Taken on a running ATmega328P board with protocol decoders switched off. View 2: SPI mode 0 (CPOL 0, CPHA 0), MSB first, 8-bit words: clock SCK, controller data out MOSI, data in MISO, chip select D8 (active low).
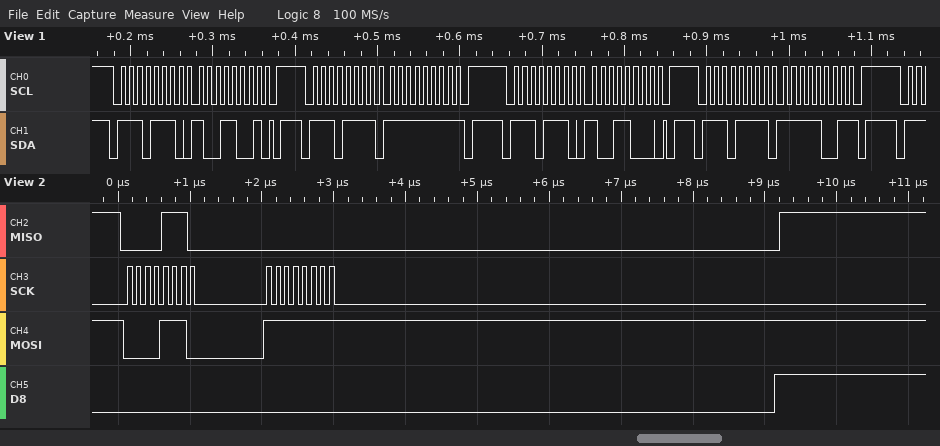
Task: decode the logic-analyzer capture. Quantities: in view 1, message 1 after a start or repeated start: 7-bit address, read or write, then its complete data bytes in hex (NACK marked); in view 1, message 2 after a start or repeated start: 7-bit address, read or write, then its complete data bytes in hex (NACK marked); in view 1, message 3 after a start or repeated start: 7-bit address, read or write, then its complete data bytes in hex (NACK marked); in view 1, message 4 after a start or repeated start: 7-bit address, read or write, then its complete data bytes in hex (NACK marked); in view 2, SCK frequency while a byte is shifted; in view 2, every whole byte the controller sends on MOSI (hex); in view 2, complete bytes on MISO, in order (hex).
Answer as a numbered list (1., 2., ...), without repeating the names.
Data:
1. 0x77 write: 99
2. 0x77 read: FF NACK
3. 0x77 write: 98
4. 0x77 read: F9 NACK
5. 8 MHz
6. 0E FF
7. 0E 00
